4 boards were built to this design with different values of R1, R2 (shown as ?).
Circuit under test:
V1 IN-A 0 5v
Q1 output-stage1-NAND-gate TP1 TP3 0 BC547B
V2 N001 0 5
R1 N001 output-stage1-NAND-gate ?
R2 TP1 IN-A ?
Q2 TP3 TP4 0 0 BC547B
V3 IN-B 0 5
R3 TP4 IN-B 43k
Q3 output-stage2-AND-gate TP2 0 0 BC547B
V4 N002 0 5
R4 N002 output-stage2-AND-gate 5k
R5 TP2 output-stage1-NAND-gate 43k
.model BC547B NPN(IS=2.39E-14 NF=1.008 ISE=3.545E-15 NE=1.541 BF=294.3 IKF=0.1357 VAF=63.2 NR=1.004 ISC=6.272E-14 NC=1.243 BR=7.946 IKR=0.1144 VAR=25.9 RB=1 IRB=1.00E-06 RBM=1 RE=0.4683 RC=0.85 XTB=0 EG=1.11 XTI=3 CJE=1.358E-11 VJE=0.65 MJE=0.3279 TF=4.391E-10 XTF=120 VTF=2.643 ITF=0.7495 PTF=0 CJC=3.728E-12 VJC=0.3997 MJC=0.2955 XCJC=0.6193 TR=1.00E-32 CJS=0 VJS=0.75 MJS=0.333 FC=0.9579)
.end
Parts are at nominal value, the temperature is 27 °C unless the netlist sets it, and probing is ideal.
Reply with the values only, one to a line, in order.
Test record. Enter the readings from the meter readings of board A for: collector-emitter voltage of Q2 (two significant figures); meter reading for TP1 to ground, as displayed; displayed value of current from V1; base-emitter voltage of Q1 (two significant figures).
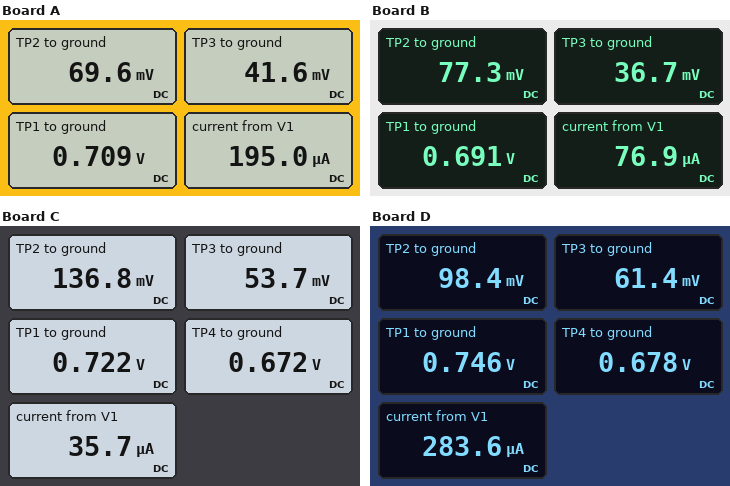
42 mV
0.709 V
195.0 µA
670 mV
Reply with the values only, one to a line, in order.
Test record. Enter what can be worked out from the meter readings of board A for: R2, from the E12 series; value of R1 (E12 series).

22 kΩ
3.3 kΩ
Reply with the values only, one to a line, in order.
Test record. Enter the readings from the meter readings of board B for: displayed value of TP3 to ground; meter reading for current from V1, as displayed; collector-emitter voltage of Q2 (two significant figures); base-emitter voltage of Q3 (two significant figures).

36.7 mV
76.9 µA
37 mV
77 mV
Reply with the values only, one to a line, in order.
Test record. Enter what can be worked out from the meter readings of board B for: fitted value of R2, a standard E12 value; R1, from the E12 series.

56 kΩ
3.9 kΩ
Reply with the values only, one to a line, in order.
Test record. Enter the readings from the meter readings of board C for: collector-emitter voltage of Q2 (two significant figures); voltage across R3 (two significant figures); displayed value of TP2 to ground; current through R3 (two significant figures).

54 mV
4.3 V
136.8 mV
100 µA
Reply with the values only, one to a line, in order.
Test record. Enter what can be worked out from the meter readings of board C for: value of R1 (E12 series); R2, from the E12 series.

1.8 kΩ
120 kΩ
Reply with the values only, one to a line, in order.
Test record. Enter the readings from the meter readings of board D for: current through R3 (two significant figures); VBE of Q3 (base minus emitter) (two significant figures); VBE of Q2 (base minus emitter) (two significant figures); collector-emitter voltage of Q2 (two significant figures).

100 µA
98 mV
680 mV
61 mV
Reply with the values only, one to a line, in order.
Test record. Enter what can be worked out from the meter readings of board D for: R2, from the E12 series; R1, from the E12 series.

15 kΩ
1.5 kΩ
